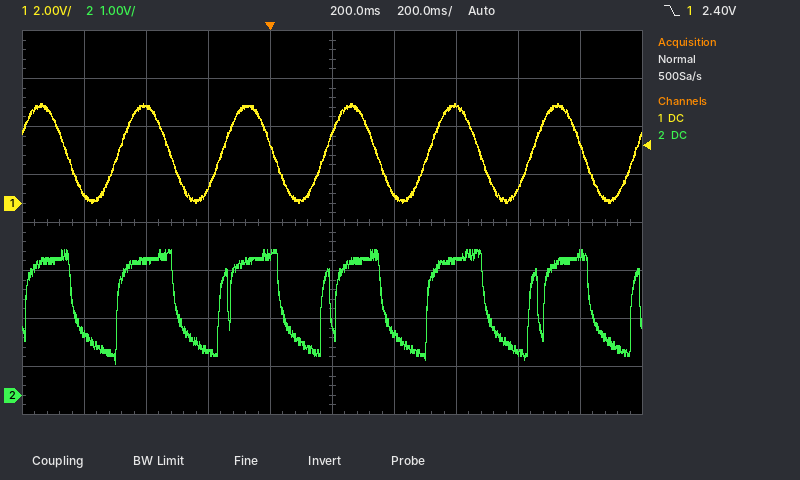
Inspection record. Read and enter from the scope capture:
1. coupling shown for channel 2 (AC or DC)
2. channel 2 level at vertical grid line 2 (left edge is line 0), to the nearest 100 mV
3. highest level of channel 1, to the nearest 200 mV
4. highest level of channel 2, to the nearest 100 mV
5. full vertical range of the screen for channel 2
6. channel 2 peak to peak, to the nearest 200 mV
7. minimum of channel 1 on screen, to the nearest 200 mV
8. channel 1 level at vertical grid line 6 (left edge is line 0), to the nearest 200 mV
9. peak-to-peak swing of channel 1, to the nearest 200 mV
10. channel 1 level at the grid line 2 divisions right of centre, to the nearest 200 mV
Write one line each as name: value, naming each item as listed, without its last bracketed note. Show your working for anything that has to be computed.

coupling shown for channel 2: DC
channel 2 level at vertical grid line 2 (left edge is line 0), to the nearest 100 mV: 2.8 V
highest level of channel 1, to the nearest 200 mV: 4.2 V
highest level of channel 2, to the nearest 100 mV: 3.0 V
full vertical range of the screen for channel 2: 8 V
channel 2 peak to peak, to the nearest 200 mV: 2.4 V
minimum of channel 1 on screen, to the nearest 200 mV: 0.0 V
channel 1 level at vertical grid line 6 (left edge is line 0), to the nearest 200 mV: 400 mV
peak-to-peak swing of channel 1, to the nearest 200 mV: 4.2 V − (0.0 V) = 4.2 V
channel 1 level at the grid line 2 divisions right of centre, to the nearest 200 mV: 4.0 V
